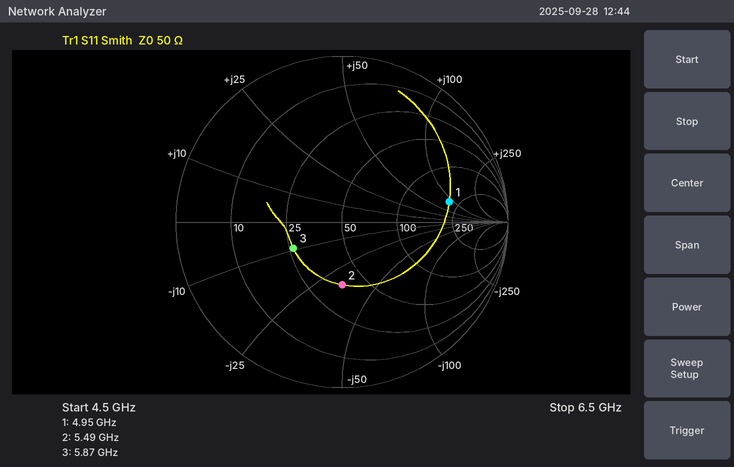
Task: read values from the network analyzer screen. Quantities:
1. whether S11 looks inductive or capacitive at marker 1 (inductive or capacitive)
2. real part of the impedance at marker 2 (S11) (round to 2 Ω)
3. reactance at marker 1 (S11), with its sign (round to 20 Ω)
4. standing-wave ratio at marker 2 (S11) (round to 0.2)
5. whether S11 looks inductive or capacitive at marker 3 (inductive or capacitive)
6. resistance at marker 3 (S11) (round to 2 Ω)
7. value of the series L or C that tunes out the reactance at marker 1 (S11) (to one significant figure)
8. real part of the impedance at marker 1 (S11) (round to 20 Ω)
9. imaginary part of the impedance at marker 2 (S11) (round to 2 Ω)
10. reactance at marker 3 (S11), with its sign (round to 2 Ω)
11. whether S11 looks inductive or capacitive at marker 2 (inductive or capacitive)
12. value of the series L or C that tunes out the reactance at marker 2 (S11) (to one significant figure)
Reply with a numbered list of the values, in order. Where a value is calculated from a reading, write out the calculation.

1. inductive
2. 38 Ω
3. +80 Ω
4. 2.2
5. capacitive
6. 26 Ω
7. C = 1/(2π × 4.95 GHz × 80 Ω) ≈ 402 fF, so 400 fF to one significant figure
8. 200 Ω
9. -34 Ω
10. -10 Ω
11. capacitive
12. L = 34 Ω/(2π × 5.49 GHz) ≈ 1.0 nH
